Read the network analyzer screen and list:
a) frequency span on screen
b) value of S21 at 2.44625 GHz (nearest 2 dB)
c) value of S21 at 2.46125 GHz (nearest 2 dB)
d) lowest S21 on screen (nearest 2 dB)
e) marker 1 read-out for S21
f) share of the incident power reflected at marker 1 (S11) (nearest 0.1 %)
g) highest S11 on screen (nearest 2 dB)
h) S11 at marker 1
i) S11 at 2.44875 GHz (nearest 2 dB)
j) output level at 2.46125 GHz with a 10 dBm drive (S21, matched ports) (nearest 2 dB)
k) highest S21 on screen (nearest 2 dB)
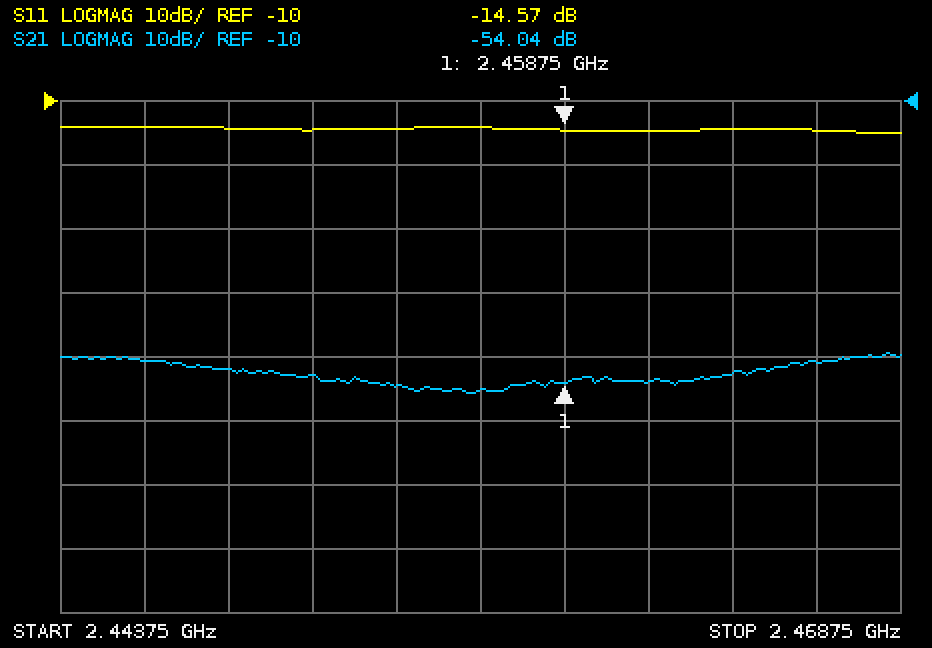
25 MHz
-50 dB
-54 dB
-56 dB
-54.04 dB
3.5 %
-14 dB
-14.57 dB
-14 dB
-44 dBm
-50 dB
